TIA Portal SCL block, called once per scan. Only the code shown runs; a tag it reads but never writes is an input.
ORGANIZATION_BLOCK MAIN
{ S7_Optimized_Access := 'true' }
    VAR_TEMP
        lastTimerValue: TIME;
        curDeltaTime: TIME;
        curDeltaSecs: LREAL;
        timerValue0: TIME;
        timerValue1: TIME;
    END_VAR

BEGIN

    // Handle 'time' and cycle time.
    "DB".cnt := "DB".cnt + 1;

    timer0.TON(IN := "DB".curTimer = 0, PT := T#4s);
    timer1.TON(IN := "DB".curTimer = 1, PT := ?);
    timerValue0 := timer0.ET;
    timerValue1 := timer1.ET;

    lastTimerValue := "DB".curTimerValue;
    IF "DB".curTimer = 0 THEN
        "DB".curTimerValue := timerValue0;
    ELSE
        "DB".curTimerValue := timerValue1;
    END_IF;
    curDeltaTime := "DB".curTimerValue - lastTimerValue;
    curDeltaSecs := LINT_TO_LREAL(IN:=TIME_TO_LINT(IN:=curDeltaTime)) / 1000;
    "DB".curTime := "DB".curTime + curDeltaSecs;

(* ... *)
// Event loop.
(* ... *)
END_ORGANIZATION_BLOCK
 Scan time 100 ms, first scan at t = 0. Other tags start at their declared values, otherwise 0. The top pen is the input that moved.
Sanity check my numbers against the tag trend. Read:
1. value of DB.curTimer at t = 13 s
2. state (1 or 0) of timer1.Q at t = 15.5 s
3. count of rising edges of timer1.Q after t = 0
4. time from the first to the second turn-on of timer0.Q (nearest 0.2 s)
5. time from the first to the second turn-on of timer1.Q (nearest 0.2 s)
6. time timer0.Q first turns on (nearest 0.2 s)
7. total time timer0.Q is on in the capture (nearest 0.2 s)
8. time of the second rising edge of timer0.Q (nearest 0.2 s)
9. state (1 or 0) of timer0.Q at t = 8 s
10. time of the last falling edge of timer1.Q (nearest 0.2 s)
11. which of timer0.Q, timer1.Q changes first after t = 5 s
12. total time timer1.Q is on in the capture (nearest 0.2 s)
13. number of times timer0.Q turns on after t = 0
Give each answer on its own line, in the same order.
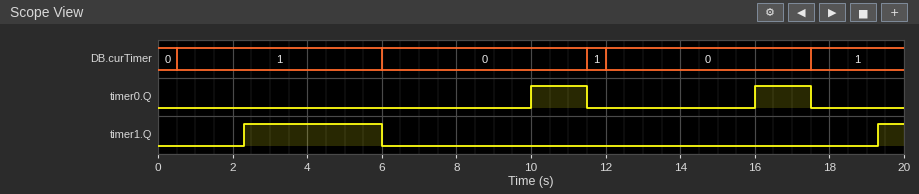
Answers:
0
0
2
6.0 s
17.0 s
10.0 s
3.0 s
16.0 s
0
6.0 s
timer1.Q
4.4 s
2
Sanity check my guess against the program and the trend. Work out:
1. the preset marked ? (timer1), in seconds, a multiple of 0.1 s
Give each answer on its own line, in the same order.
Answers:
1.8 s
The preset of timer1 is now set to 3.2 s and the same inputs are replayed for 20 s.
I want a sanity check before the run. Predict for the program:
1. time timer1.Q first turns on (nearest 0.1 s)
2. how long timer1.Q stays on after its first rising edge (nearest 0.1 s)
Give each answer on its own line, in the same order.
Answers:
3.7 s
2.3 s
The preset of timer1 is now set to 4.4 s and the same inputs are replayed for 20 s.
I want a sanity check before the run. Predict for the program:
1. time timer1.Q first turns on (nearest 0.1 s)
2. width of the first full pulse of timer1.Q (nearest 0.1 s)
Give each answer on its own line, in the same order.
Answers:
4.9 s
1.1 s
